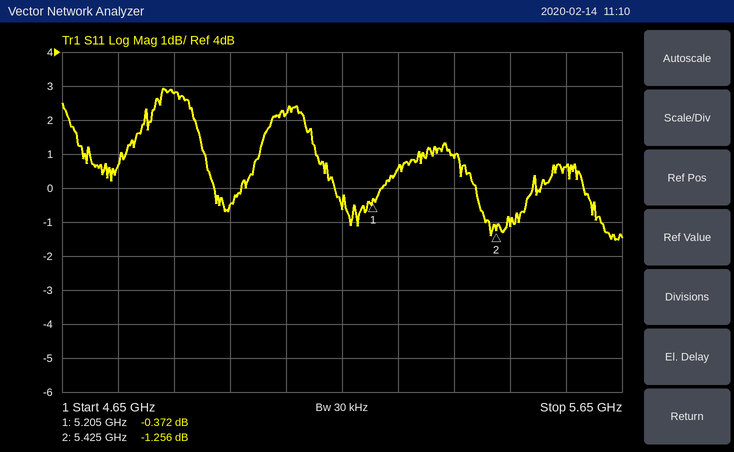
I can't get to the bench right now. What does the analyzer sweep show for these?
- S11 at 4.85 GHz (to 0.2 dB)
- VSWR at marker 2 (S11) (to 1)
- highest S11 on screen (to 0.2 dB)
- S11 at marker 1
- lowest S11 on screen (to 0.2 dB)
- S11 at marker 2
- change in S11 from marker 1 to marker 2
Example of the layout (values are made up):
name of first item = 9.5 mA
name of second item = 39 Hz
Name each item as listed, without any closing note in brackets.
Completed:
S11 at 4.85 GHz = 2.8 dB
VSWR at marker 2 (S11) = 14
highest S11 on screen = 3.0 dB
S11 at marker 1 = -0.372 dB
lowest S11 on screen = -1.6 dB
S11 at marker 2 = -1.256 dB
change in S11 from marker 1 to marker 2 = -0.884 dB
